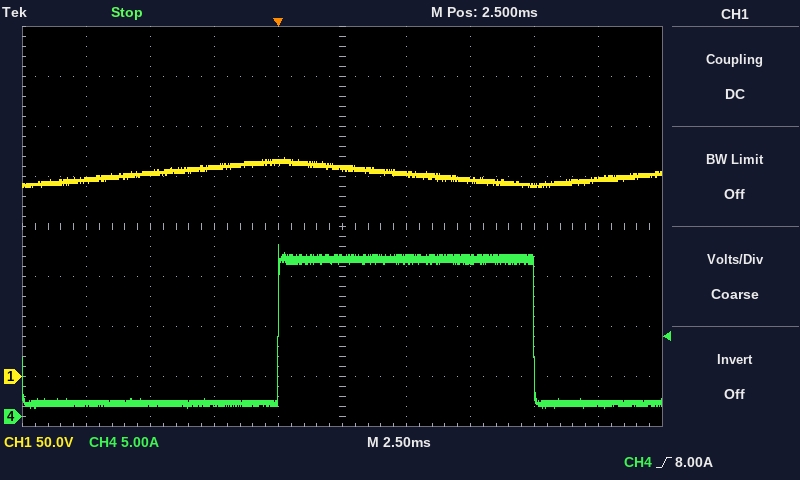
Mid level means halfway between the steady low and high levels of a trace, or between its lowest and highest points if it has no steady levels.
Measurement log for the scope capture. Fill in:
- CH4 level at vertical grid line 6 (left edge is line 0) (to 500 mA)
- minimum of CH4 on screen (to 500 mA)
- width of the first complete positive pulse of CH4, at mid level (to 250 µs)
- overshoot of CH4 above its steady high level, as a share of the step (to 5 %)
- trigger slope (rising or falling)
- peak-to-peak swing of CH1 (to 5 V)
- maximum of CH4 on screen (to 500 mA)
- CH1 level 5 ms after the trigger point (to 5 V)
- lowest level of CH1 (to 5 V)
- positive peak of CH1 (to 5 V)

15.5 A
1.0 A
10.00 ms
10 %
rising
30 V
17.0 A
200 V
190 V
220 V
